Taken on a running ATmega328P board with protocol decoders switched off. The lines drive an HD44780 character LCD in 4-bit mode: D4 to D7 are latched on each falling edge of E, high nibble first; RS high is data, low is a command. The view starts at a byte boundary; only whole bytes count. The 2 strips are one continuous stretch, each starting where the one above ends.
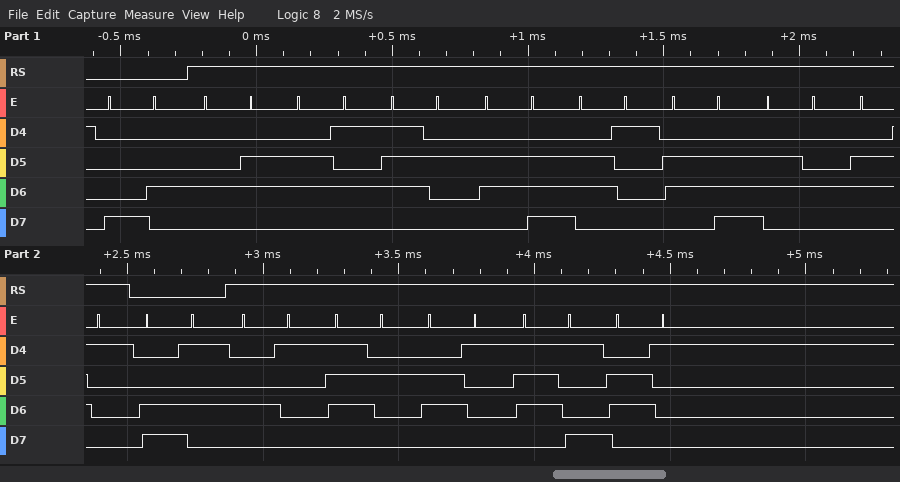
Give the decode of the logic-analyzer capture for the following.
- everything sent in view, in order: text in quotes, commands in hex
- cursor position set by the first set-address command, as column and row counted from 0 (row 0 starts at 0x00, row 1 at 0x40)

0x84 "Fernanda" 0xC5 "Araya"
column 4, row 0
